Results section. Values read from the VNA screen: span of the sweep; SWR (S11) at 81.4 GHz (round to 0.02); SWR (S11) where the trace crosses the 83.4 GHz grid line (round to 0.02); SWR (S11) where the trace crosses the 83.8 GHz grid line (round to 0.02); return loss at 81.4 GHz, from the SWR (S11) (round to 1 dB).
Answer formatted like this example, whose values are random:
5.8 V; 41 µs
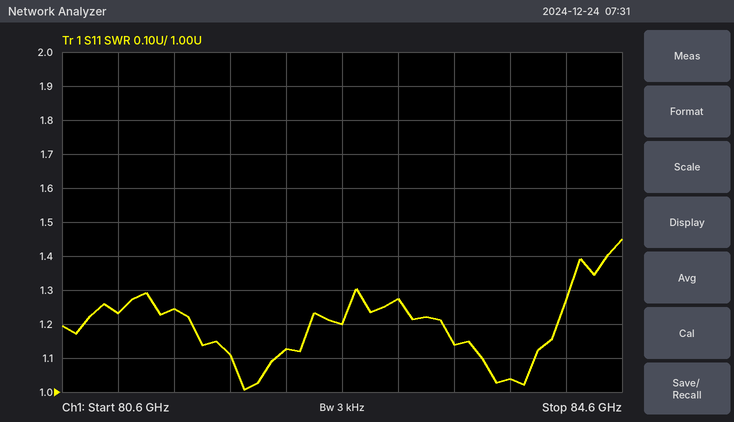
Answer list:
4 GHz; 1.24; 1.14; 1.04; 19 dB
